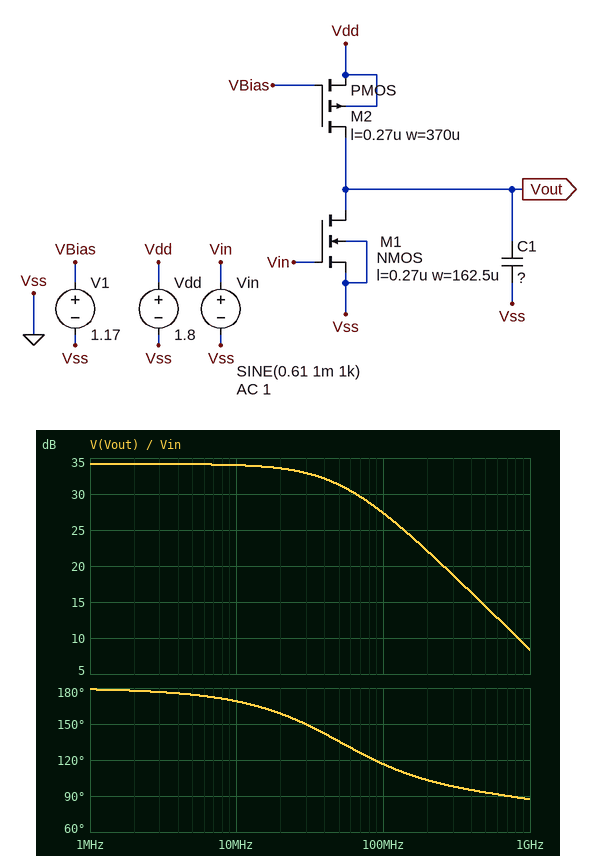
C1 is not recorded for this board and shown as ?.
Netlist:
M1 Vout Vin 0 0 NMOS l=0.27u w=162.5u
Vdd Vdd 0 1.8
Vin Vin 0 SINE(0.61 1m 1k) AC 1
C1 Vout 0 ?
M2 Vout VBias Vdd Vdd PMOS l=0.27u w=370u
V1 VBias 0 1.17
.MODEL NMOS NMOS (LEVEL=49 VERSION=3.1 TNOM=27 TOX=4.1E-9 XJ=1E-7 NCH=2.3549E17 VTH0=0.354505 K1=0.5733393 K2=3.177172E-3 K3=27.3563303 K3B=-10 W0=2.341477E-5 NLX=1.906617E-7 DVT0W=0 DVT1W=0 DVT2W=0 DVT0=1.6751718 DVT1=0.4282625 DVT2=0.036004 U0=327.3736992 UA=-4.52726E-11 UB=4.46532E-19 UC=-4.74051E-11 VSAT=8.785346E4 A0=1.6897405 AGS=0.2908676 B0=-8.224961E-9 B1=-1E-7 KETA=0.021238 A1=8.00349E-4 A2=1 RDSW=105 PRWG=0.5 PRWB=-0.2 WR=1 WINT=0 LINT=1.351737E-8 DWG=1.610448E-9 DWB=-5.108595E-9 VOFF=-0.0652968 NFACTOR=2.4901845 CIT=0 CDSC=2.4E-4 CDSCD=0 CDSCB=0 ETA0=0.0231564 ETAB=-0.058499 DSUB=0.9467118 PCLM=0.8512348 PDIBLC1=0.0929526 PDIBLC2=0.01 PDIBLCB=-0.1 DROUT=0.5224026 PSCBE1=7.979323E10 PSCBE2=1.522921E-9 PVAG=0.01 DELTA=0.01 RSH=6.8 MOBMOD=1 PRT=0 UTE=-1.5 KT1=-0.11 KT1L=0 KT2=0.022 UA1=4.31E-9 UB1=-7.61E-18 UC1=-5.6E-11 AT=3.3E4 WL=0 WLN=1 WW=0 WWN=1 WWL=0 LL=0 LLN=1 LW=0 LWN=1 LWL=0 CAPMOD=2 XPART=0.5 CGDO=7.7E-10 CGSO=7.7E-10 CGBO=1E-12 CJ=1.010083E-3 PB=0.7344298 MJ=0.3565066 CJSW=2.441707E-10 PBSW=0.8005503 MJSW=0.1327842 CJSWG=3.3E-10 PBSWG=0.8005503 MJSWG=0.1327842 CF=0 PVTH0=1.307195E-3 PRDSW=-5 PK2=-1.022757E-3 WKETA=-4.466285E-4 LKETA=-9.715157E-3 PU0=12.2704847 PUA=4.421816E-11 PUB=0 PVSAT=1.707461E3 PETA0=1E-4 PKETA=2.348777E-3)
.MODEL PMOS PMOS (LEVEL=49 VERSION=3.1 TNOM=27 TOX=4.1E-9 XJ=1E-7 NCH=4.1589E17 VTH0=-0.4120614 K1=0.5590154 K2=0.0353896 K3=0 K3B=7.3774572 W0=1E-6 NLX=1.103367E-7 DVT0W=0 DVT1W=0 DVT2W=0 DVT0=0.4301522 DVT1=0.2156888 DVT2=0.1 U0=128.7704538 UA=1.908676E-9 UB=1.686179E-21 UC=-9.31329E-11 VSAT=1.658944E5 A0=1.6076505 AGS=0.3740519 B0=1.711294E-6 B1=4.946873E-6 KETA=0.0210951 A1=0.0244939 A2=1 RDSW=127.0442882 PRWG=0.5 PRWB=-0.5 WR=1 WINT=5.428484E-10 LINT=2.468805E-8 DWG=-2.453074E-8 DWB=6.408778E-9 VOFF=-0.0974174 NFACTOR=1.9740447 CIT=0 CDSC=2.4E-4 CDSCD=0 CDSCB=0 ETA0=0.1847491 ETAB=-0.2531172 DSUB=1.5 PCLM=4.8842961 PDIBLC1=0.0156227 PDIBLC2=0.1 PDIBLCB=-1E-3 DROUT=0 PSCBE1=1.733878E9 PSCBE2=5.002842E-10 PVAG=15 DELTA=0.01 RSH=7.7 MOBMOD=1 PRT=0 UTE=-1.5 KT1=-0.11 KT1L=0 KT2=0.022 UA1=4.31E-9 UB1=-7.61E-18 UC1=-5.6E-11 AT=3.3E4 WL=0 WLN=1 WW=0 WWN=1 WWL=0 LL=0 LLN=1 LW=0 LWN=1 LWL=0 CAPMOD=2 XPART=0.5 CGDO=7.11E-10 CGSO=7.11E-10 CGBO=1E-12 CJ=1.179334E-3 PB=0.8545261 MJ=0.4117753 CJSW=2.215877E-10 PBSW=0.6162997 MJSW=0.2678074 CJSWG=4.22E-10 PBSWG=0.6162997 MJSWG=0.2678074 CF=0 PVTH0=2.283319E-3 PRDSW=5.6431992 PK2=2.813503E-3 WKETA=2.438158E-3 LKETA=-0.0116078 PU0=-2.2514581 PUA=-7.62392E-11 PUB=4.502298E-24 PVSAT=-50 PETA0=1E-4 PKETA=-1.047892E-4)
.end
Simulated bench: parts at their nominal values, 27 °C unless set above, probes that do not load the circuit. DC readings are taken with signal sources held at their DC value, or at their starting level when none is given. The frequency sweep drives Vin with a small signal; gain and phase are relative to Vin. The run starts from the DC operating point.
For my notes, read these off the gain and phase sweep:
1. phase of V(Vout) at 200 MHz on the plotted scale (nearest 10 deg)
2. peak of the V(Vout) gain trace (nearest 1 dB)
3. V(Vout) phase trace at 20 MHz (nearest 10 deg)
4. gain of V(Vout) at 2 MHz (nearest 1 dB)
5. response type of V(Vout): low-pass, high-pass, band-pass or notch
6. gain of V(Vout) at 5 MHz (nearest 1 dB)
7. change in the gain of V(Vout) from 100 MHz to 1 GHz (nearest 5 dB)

100 deg
34 dB
160 deg
34 dB
low-pass
34 dB
-20 dB
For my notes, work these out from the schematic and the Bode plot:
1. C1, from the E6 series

330 fF
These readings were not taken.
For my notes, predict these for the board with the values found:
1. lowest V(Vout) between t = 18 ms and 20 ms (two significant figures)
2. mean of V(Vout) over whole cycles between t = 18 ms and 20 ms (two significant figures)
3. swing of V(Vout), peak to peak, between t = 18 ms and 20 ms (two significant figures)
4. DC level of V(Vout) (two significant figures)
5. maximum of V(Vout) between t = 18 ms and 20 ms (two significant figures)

1.1 V
1.1 V
100 mV
1.1 V
1.2 V
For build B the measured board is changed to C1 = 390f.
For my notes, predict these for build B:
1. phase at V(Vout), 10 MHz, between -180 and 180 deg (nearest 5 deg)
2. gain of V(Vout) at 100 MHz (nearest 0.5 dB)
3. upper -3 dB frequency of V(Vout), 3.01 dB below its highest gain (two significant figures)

170 deg
27.0 dB
48 MHz
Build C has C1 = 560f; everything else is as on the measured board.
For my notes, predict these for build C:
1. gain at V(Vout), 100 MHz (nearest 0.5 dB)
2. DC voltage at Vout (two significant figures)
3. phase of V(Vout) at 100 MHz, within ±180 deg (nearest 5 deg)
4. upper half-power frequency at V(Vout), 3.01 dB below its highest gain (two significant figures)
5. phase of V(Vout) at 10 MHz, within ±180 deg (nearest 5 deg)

25.5 dB
1.1 V
110 deg
41 MHz
165 deg
